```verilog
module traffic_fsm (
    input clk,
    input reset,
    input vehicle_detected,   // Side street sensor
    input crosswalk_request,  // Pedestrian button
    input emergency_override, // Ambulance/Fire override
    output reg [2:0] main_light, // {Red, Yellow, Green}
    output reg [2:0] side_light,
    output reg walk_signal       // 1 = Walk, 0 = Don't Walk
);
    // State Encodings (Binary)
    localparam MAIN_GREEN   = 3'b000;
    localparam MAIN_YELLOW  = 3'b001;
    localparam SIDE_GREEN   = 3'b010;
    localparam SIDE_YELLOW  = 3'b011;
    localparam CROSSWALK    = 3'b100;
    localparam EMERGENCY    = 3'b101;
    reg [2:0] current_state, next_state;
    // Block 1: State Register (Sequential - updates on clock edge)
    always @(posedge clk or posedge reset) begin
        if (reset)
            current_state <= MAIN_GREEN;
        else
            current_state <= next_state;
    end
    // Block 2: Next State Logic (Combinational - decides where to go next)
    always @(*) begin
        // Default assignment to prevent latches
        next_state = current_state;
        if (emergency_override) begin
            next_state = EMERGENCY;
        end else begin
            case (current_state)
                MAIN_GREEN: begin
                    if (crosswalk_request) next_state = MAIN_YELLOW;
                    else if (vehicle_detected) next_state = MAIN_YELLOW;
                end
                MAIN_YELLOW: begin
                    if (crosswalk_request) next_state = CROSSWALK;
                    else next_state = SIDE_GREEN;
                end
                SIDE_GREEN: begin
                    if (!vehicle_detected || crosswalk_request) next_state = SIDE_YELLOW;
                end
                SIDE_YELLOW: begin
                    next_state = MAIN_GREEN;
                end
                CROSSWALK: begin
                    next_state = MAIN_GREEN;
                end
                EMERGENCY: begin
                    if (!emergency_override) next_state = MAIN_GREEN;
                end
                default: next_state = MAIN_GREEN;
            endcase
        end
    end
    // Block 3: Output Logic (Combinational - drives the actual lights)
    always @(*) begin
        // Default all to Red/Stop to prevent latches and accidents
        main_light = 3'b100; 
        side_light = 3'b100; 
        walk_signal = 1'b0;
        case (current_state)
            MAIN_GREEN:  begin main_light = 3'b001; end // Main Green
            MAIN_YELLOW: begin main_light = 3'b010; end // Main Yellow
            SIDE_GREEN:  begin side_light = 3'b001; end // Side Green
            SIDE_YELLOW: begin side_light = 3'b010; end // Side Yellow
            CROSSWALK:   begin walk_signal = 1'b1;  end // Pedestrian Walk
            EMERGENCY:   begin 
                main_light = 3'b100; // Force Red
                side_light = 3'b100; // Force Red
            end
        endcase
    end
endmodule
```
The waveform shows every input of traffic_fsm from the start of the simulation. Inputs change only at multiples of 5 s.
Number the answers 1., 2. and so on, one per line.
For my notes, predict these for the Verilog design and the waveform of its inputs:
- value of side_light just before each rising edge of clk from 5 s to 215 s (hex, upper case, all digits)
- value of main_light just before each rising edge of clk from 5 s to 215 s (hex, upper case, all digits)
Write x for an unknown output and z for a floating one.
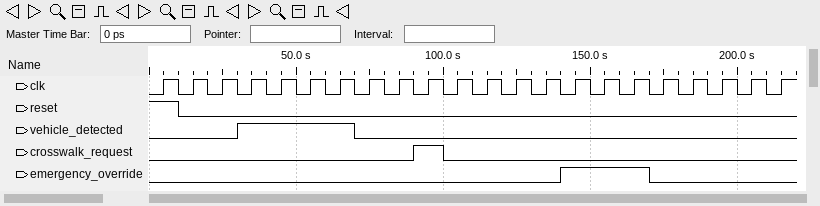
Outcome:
1. 4, 4, 4, 4, 4, 1, 1, 1, 2, 4, 4, 1, 2, 4, 4, 4, 4, 4, 4, 4, 4, 4
2. 1, 1, 1, 1, 2, 4, 4, 4, 4, 1, 2, 4, 4, 1, 1, 4, 4, 4, 1, 1, 1, 1
